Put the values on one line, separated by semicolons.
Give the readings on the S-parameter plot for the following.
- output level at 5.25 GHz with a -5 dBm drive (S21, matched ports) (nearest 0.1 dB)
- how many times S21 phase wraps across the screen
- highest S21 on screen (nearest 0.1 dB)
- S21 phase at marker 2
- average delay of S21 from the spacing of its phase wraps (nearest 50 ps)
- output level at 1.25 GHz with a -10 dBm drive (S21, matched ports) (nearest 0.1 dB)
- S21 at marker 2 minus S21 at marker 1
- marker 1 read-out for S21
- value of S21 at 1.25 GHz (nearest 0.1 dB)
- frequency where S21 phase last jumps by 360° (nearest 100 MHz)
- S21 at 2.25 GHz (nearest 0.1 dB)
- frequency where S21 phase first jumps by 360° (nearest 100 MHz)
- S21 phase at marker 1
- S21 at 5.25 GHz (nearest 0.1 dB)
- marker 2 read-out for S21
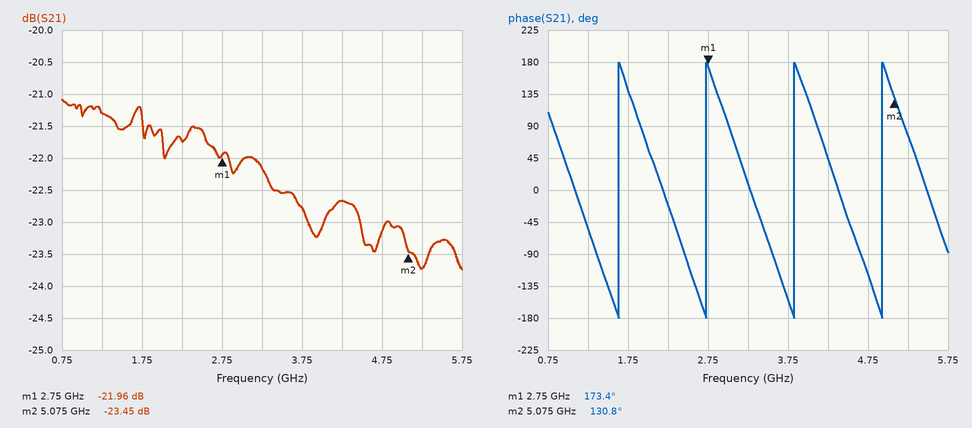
-28.7 dBm; 4; -21.1 dB; 130.8°; 900 ps; -31.3 dBm; -1.49 dB; -21.96 dB; -21.3 dB; 4.9 GHz; -21.7 dB; 1.6 GHz; 173.4°; -23.7 dB; -23.45 dB
